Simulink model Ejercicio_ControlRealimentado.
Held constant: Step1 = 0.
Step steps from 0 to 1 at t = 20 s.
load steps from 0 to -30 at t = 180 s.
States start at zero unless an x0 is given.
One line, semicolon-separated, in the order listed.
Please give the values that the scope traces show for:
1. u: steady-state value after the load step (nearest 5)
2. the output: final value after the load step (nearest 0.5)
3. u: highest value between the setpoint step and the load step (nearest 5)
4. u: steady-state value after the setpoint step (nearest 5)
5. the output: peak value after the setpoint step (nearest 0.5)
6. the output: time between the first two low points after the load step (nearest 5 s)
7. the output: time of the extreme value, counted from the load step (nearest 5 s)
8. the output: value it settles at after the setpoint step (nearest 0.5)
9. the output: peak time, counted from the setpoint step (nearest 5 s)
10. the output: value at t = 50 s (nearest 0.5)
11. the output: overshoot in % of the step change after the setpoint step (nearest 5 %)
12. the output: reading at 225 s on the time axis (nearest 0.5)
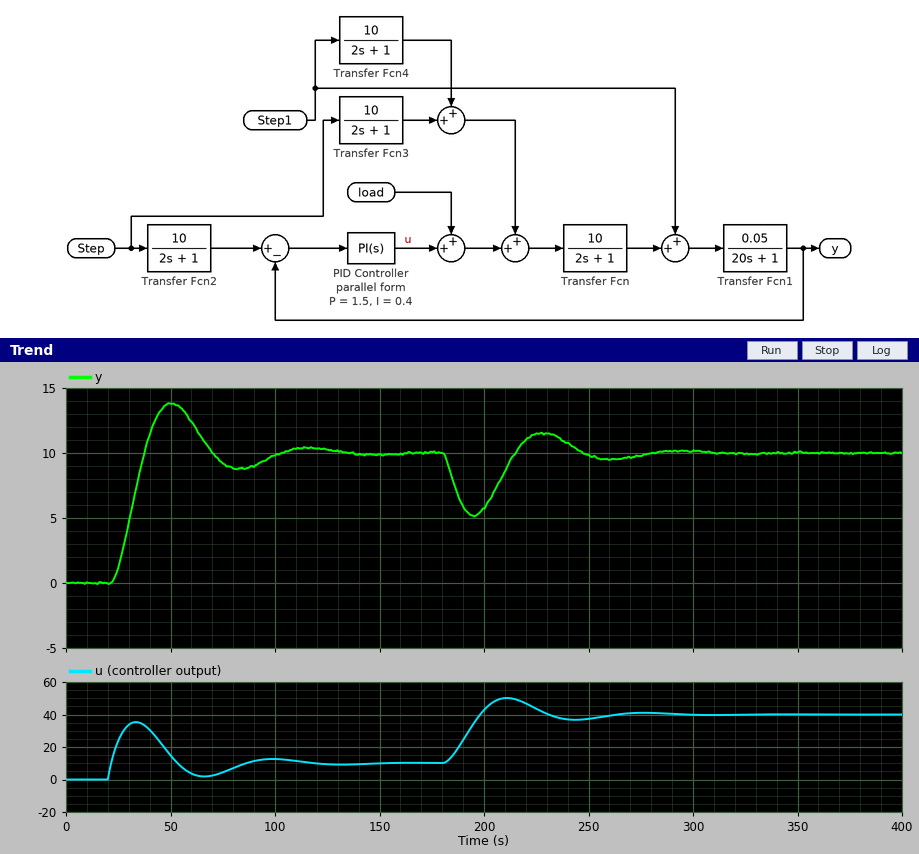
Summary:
40; 10.0; 35; 10; 14.0; 65 s; 15 s; 10.0; 30 s; 14.0; 40 %; 11.5
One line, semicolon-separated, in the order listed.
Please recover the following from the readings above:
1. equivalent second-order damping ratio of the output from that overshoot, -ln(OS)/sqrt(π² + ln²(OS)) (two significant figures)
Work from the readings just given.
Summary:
0.28
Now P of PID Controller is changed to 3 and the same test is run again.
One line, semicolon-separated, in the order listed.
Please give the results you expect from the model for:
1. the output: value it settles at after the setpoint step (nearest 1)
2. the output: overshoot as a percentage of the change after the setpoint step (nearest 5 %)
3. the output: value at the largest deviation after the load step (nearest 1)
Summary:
10; 25 %; 6
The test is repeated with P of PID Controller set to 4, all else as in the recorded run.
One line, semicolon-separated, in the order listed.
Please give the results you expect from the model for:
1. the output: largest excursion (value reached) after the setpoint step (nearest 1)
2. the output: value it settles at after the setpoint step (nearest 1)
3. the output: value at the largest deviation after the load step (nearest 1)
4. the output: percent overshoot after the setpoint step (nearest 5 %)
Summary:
12; 10; 6; 20 %
